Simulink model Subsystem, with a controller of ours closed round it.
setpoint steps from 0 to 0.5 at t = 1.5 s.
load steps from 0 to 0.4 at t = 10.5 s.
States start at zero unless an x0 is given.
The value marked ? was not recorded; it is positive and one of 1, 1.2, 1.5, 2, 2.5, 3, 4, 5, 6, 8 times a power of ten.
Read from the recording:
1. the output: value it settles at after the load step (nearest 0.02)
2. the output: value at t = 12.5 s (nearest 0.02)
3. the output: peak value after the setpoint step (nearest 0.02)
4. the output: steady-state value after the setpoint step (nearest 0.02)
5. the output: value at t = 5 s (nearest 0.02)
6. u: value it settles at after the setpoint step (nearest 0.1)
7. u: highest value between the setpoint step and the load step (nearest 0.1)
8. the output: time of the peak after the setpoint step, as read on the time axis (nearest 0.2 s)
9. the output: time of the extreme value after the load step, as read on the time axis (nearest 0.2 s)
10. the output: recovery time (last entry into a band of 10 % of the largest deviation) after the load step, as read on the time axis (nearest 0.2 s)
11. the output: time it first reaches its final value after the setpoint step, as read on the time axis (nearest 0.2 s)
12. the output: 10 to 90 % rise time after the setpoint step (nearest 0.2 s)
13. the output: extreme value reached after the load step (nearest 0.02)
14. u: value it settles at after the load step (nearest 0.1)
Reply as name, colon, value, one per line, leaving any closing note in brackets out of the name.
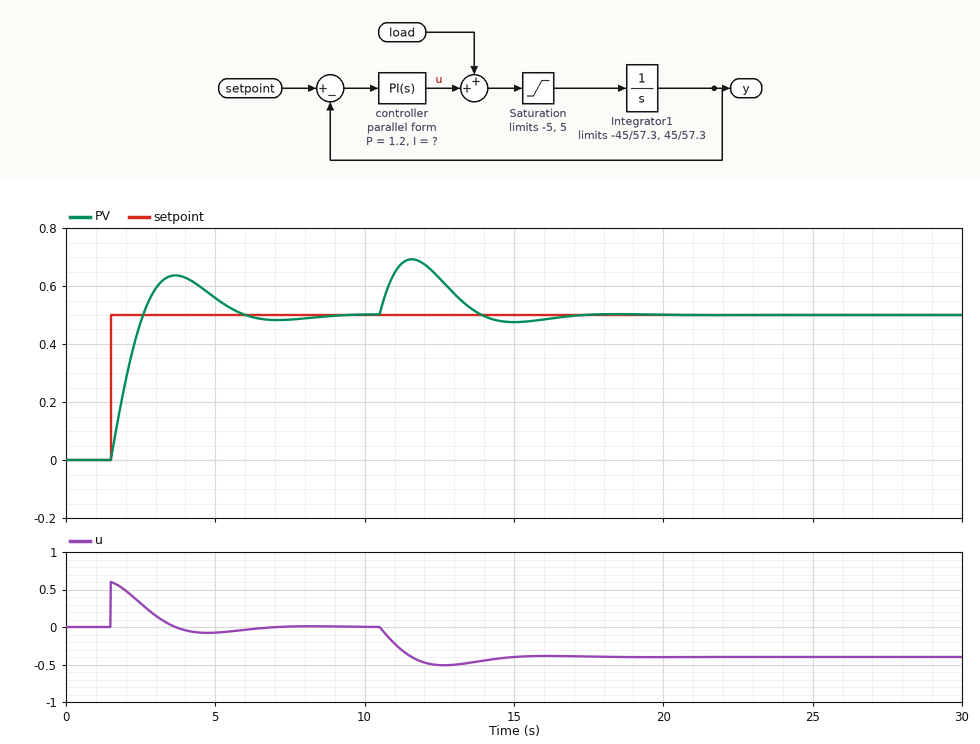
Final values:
the output: value it settles at after the load step: 0.50
the output: value at t = 12.5 s: 0.62
the output: peak value after the setpoint step: 0.64
the output: steady-state value after the setpoint step: 0.50
the output: value at t = 5 s: 0.56
u: value it settles at after the setpoint step: 0.0
u: highest value between the setpoint step and the load step: 0.6
the output: time of the peak after the setpoint step, as read on the time axis: 3.6 s
the output: time of the extreme value after the load step, as read on the time axis: 11.6 s
the output: recovery time (last entry into a band of 10 % of the largest deviation) after the load step, as read on the time axis: 15.8 s
the output: time it first reaches its final value after the setpoint step, as read on the time axis: 2.6 s
the output: 10 to 90 % rise time after the setpoint step: 0.8 s
the output: extreme value reached after the load step: 0.70
u: value it settles at after the load step: -0.4
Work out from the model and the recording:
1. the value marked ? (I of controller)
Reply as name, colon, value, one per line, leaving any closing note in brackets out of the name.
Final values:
the value marked ?: 1.2
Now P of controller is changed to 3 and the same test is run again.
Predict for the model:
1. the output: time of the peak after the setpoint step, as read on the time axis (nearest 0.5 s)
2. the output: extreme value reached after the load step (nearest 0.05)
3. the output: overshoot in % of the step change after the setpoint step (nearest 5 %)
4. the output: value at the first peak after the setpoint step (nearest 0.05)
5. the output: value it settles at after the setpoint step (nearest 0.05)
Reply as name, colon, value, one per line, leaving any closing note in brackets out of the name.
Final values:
the output: time of the peak after the setpoint step, as read on the time axis: 3.0 s
the output: extreme value reached after the load step: 0.60
the output: overshoot in % of the step change after the setpoint step: 10 %
the output: value at the first peak after the setpoint step: 0.55
the output: value it settles at after the setpoint step: 0.50
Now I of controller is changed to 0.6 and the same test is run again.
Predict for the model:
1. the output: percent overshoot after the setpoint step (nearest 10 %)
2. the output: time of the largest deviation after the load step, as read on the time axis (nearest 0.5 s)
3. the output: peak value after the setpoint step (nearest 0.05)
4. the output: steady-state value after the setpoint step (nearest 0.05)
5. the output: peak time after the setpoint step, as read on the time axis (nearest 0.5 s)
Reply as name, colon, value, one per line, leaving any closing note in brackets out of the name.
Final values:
the output: percent overshoot after the setpoint step: 20 %
the output: time of the largest deviation after the load step, as read on the time axis: 12.0 s
the output: peak value after the setpoint step: 0.60
the output: steady-state value after the setpoint step: 0.50
the output: peak time after the setpoint step, as read on the time axis: 4.5 s
